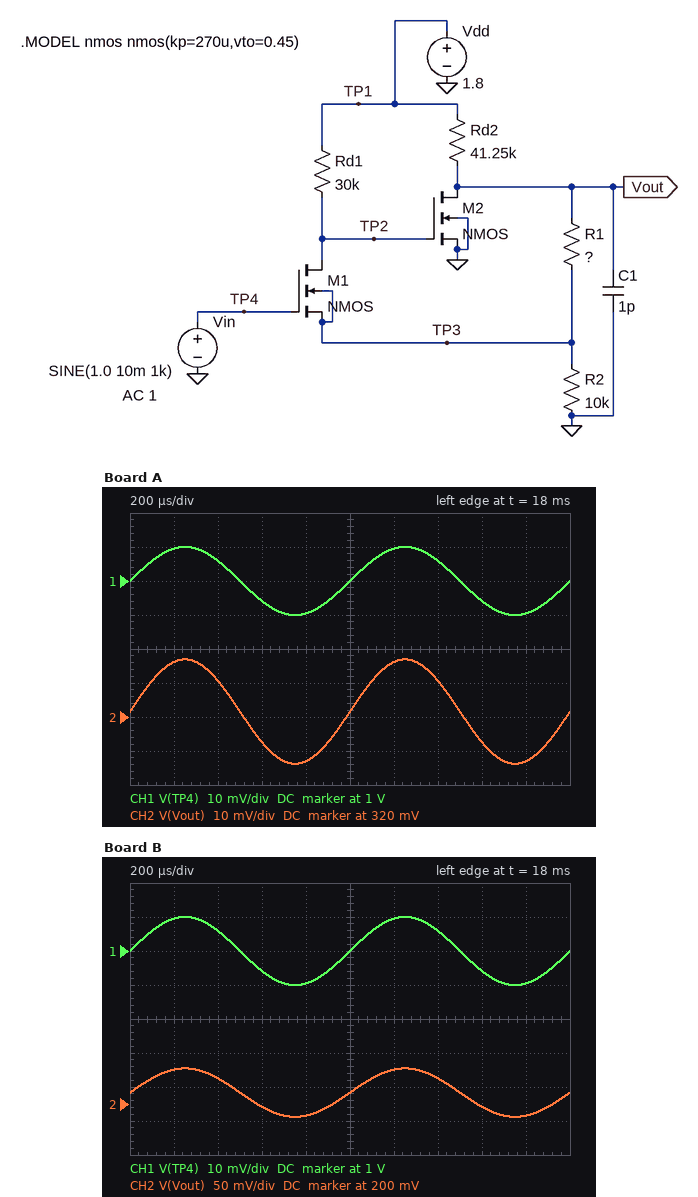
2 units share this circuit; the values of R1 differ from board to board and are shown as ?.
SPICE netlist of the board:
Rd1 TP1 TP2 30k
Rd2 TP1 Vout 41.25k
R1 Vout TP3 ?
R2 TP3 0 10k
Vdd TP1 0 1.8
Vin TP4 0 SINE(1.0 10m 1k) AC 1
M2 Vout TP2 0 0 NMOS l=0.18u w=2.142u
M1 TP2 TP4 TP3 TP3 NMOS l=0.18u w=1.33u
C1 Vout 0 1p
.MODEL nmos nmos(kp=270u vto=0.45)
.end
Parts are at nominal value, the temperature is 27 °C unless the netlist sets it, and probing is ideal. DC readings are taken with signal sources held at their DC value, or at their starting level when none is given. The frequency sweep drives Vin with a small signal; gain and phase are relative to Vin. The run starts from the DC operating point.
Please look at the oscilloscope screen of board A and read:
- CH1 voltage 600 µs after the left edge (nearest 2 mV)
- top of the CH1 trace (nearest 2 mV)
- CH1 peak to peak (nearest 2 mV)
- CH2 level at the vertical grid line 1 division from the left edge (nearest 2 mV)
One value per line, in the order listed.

994 mV
1.010 V
20 mV
336 mV
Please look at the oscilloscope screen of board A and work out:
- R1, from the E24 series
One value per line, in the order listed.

6.2 kΩ
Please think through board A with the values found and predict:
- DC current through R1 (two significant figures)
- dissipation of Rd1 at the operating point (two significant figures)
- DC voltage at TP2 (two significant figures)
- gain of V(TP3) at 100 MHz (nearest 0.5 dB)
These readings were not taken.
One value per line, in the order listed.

4.7 µA
47 µW
610 mV
-0.5 dB
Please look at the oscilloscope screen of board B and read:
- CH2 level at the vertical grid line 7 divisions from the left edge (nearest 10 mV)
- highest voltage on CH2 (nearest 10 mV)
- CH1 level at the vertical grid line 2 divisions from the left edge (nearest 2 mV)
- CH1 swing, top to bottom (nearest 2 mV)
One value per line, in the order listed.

240 mV
250 mV
1.006 V
20 mV
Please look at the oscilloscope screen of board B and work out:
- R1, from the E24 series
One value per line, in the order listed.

30 kΩ
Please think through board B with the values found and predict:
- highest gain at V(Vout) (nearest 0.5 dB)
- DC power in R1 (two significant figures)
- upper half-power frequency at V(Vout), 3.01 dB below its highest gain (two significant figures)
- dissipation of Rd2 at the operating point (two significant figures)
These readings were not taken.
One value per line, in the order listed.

11.0 dB
600 nW
71 MHz
61 µW
